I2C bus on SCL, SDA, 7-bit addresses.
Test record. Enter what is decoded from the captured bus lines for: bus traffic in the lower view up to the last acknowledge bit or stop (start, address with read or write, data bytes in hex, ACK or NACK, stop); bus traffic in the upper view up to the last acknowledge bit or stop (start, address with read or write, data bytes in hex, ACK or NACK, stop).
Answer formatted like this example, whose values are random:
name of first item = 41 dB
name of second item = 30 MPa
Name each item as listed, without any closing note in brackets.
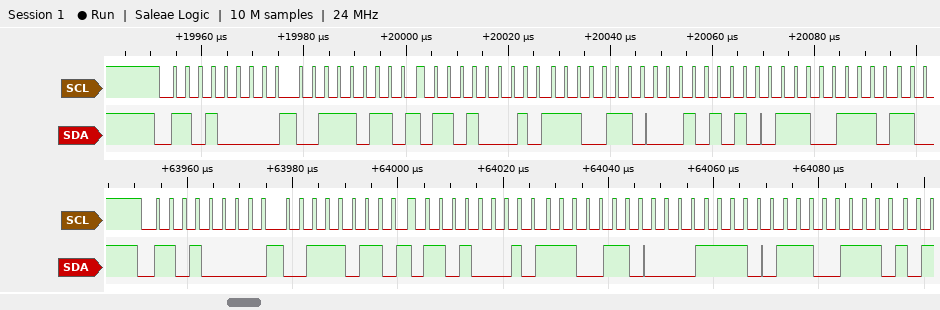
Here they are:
bus traffic in the lower view up to the last acknowledge bit or stop = start, address 68 write ACK, 3B ACK, repeated start, address 68 read ACK, E6 ACK, 1E ACK, E7 ACK
bus traffic in the upper view up to the last acknowledge bit or stop = start, address 68 write ACK, 3B ACK, repeated start, address 68 read ACK, E6 ACK, 2A ACK, E7 ACK
